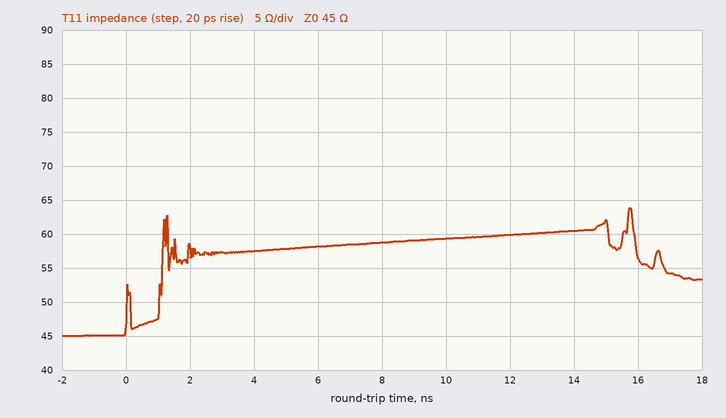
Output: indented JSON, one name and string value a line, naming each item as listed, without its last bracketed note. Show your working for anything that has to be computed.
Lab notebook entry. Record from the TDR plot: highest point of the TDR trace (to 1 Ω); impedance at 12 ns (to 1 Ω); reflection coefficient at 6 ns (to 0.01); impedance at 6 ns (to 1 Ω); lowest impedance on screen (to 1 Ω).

{
  "highest point of the TDR trace": "64 Ω",
  "impedance at 12 ns": "60 Ω",
  "reflection coefficient at 6 ns": "(58 − 45)/(58 + 45) ≈ +0.13",
  "impedance at 6 ns": "58 Ω",
  "lowest impedance on screen": "45 Ω"
}
